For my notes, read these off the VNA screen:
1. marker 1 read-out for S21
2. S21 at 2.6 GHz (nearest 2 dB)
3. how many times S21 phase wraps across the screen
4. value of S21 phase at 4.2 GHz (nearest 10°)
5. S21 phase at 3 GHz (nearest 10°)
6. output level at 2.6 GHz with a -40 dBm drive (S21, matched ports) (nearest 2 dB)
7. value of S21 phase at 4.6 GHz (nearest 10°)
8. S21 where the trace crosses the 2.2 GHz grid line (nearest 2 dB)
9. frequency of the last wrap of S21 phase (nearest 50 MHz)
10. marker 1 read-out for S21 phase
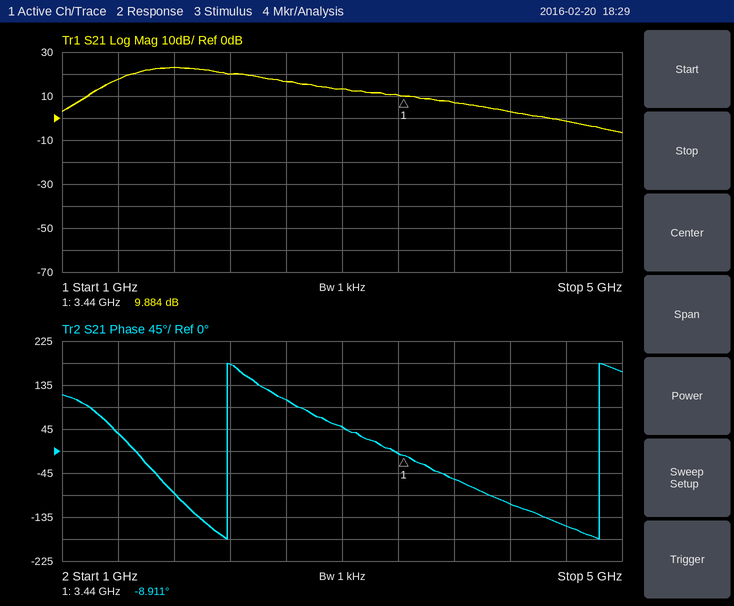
9.884 dB
16 dB
2
-110°
50°
-24 dBm
-150°
20 dB
4.85 GHz
-8.911°
